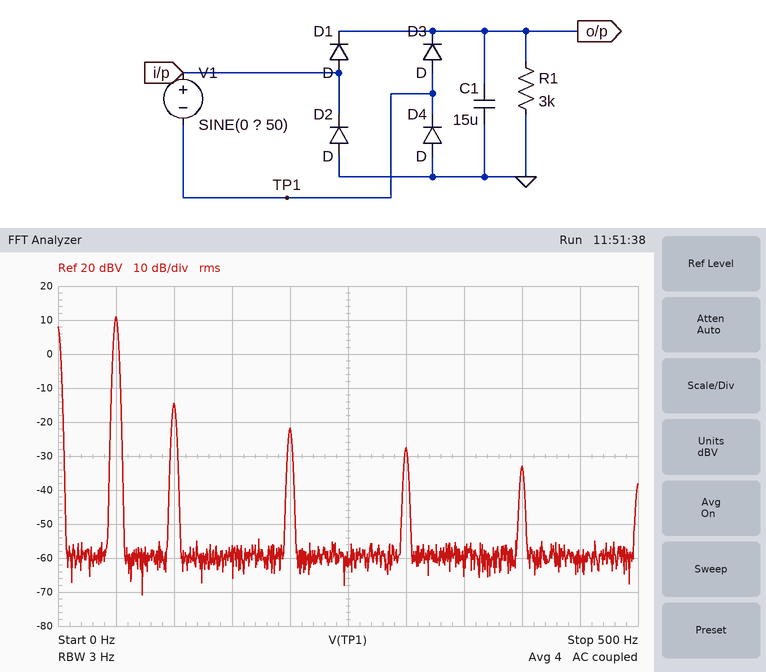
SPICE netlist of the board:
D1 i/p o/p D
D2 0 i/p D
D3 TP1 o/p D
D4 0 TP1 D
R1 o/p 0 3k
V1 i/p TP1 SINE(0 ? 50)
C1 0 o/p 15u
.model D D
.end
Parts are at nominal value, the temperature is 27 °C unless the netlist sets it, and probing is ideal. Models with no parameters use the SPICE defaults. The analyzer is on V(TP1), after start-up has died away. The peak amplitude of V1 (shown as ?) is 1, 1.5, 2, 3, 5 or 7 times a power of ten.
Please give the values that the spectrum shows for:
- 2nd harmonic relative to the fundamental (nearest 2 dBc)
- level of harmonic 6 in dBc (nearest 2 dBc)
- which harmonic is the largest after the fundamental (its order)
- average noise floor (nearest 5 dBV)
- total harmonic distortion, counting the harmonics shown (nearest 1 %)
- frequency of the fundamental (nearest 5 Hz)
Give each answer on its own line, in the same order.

-26 dBc
-38 dBc
2
-60 dBV
6 %
50 Hz
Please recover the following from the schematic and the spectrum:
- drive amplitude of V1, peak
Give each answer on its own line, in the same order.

10 V
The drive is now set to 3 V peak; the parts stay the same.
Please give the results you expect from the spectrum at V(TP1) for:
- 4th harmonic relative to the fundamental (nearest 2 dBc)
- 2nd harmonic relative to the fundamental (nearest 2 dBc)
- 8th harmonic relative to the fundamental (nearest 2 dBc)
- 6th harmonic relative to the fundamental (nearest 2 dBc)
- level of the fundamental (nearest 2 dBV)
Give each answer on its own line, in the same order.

-36 dBc
-30 dBc
-48 dBc
-42 dBc
0 dBV
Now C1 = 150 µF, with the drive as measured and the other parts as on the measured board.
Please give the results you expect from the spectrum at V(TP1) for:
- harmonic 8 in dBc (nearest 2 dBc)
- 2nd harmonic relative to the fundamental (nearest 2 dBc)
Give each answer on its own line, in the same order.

-58 dBc
-44 dBc
